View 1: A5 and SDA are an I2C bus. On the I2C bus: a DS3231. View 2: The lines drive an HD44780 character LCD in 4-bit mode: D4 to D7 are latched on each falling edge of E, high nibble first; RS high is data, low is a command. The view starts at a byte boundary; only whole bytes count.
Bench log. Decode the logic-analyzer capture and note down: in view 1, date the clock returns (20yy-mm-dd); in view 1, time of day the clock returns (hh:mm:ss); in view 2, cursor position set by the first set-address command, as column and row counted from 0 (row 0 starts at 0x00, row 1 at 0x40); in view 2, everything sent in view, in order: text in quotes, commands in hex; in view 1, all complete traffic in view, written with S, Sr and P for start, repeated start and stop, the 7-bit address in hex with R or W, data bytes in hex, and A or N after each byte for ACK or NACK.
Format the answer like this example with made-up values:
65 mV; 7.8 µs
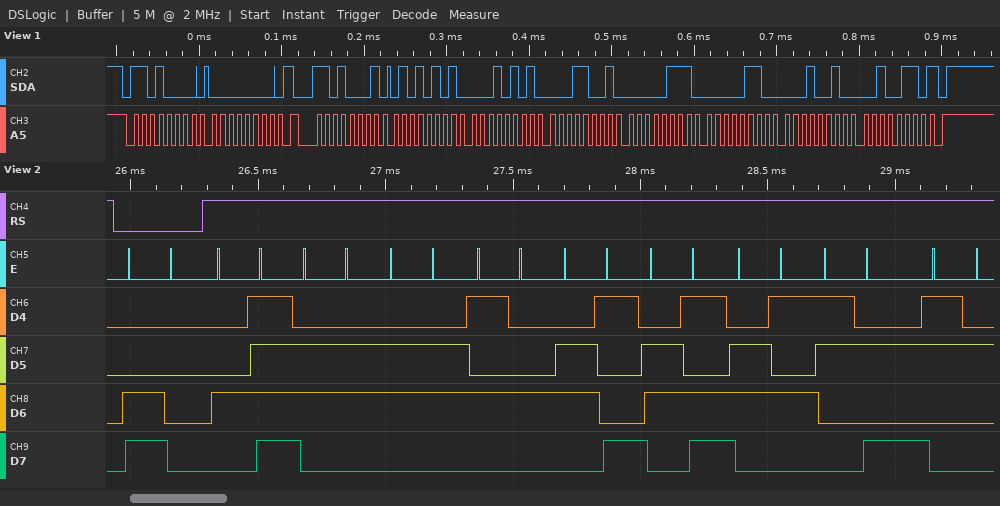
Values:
2026-12-06; 19:15:55; column 0, row 1; 0xC0 "OffTime:2"; S 68W A 00 A Sr 68R A 55 A 15 A 19 A 07 A 06 A 12 A 26 N P
